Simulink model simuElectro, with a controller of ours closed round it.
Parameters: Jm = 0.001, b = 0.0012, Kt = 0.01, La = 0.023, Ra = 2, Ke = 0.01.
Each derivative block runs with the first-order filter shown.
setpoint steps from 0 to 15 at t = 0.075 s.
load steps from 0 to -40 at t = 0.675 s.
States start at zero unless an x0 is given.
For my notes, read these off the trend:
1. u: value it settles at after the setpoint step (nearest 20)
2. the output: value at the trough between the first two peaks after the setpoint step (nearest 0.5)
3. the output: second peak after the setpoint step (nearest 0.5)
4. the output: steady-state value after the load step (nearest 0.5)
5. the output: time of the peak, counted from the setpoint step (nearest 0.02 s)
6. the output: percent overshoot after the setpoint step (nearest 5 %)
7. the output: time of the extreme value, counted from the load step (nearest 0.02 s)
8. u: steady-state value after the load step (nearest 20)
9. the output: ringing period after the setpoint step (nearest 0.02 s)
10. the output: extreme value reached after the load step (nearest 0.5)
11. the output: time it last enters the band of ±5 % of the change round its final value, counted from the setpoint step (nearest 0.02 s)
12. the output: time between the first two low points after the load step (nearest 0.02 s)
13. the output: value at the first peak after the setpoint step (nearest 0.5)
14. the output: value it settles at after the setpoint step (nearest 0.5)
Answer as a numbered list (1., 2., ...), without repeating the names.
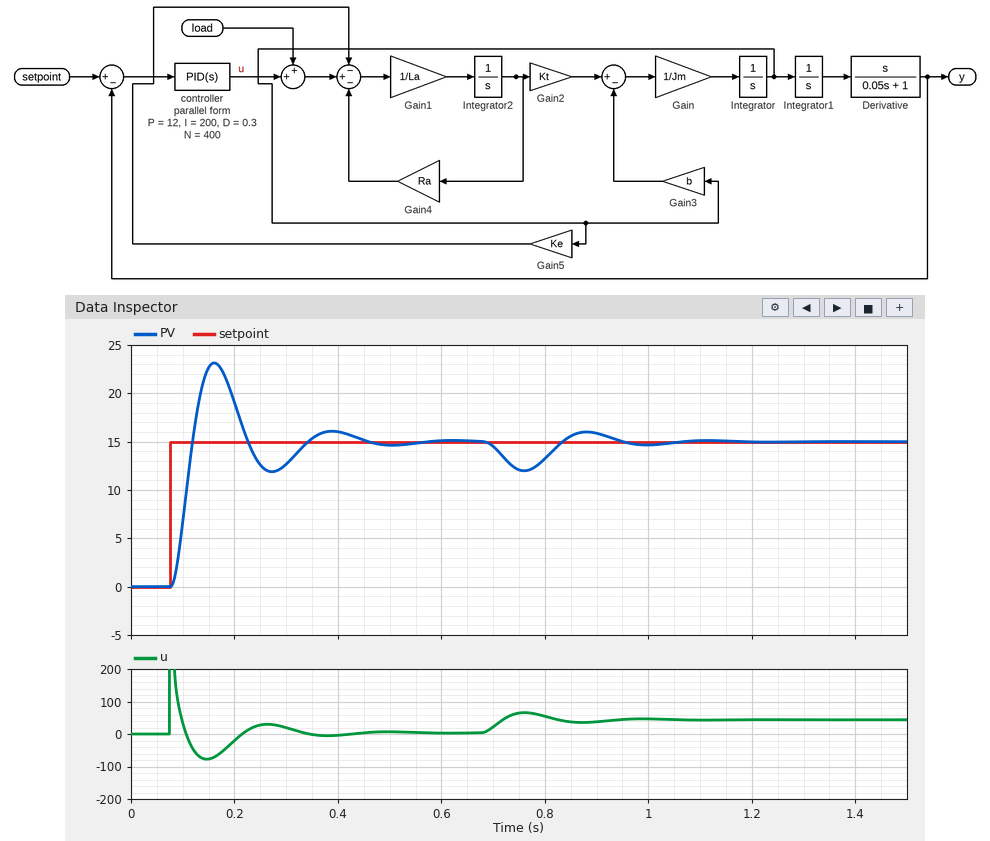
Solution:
1. 0
2. 12.0
3. 16.0
4. 15.0
5. 0.08 s
6. 55 %
7. 0.08 s
8. 40
9. 0.22 s
10. 12.0
11. 0.34 s
12. 0.24 s
13. 23.0
14. 15.0
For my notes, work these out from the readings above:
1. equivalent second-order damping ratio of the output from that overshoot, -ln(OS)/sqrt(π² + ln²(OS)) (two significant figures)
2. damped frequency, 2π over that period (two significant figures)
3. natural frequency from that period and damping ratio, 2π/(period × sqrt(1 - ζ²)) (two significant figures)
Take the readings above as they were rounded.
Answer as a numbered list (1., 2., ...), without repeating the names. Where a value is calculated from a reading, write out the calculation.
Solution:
1. ln(0.55) = -0.598; 0.598 / sqrt(9.870 + 0.357) = 0.19
2. 2π / 0.22 = 29 rad/s
3. 2π / (0.22 × sqrt(1 - 0.19²)) = 29 rad/s
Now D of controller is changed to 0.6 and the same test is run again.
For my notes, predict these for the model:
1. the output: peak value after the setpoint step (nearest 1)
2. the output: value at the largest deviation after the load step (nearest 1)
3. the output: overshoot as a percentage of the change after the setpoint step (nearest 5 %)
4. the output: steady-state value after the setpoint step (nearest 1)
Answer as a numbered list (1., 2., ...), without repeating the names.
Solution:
1. 19
2. 13
3. 25 %
4. 15
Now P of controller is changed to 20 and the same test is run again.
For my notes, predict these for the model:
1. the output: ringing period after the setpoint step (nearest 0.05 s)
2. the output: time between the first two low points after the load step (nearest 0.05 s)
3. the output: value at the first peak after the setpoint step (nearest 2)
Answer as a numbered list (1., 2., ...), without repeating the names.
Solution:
1. 0.15 s
2. 0.15 s
3. 24
